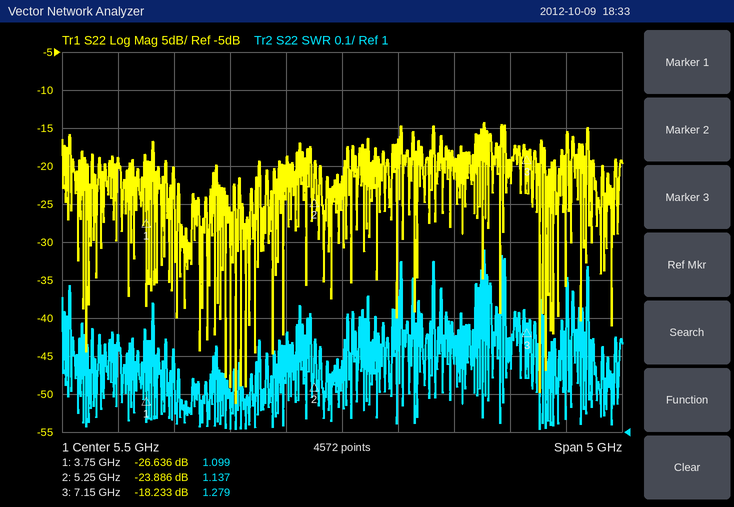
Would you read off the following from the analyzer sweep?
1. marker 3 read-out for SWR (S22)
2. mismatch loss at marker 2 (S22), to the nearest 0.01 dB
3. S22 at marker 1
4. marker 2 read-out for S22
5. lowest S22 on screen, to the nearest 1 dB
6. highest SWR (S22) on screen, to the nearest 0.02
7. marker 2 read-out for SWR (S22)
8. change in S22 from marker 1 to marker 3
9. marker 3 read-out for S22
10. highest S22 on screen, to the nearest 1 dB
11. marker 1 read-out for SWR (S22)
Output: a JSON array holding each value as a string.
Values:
["1.279", "0.02 dB", "-26.636 dB", "-23.886 dB", "-51 dB", "1.48", "1.137", "8.403 dB", "-18.233 dB", "-14 dB", "1.099"]
